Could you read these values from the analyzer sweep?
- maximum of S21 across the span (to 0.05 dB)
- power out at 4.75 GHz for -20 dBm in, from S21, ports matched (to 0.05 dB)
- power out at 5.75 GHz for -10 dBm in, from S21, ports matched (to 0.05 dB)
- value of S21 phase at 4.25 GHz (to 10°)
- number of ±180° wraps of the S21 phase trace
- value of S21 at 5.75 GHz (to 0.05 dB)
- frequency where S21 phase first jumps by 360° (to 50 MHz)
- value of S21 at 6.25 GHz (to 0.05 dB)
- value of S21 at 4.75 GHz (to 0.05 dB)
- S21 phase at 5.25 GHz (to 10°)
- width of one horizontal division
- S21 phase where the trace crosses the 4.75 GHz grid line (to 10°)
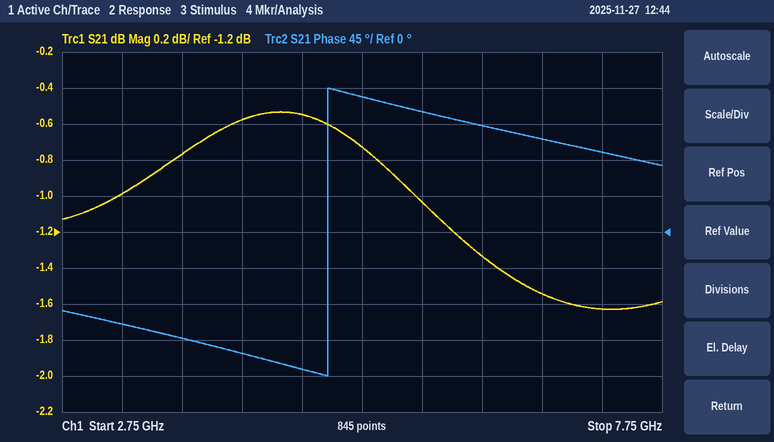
-0.55 dB
-20.55 dBm
-11.05 dBm
-150°
1
-1.05 dB
4.95 GHz
-1.35 dB
-0.55 dB
170°
500 MHz
-170°
